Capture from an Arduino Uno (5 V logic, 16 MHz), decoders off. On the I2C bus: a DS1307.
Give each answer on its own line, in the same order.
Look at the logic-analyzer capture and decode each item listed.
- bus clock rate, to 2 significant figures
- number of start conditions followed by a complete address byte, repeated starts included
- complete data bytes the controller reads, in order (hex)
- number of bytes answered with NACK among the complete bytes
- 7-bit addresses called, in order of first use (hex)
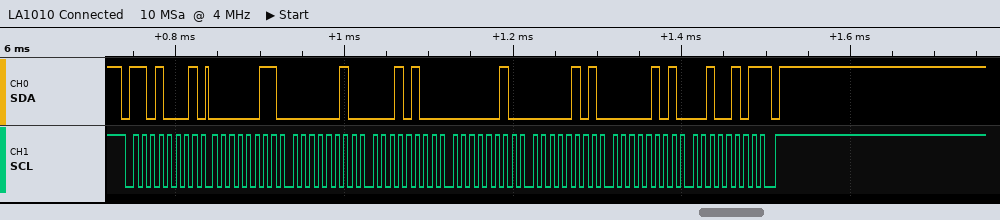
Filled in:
100 kHz
1
03 02 14 02 05 05 25
1
0x68
